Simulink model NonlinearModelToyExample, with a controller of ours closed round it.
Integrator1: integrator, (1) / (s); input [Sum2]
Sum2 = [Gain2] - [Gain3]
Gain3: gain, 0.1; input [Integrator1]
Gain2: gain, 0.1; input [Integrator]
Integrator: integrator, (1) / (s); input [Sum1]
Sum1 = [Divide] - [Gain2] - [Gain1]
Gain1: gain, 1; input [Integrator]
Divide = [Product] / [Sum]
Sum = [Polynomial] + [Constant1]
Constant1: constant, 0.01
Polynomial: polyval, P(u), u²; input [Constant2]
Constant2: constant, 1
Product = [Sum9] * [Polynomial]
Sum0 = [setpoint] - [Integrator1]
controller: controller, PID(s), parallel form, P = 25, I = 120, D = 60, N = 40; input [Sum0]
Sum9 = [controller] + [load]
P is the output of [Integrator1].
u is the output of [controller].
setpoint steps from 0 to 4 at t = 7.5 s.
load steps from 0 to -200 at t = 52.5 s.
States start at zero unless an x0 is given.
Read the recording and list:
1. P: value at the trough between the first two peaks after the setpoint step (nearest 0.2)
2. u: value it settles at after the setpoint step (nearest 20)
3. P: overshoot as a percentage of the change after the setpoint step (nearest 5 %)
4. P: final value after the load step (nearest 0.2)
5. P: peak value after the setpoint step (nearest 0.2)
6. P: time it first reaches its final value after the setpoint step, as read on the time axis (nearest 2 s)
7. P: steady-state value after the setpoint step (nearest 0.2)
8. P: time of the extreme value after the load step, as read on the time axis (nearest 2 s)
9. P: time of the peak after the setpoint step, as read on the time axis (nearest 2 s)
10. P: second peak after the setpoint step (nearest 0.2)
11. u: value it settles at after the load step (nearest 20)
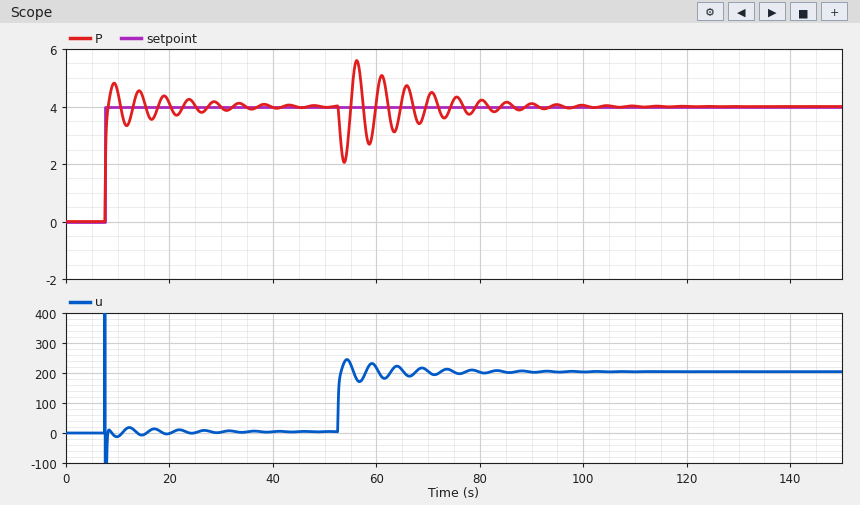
3.4
0
20 %
4.0
4.8
8 s
4.0
54 s
10 s
4.6
200
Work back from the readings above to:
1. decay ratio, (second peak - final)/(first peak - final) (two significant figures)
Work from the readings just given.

0.75
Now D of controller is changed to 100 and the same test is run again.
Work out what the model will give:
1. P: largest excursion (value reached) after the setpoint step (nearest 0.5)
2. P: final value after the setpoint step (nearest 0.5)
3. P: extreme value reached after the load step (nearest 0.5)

4.5
4.0
2.5
